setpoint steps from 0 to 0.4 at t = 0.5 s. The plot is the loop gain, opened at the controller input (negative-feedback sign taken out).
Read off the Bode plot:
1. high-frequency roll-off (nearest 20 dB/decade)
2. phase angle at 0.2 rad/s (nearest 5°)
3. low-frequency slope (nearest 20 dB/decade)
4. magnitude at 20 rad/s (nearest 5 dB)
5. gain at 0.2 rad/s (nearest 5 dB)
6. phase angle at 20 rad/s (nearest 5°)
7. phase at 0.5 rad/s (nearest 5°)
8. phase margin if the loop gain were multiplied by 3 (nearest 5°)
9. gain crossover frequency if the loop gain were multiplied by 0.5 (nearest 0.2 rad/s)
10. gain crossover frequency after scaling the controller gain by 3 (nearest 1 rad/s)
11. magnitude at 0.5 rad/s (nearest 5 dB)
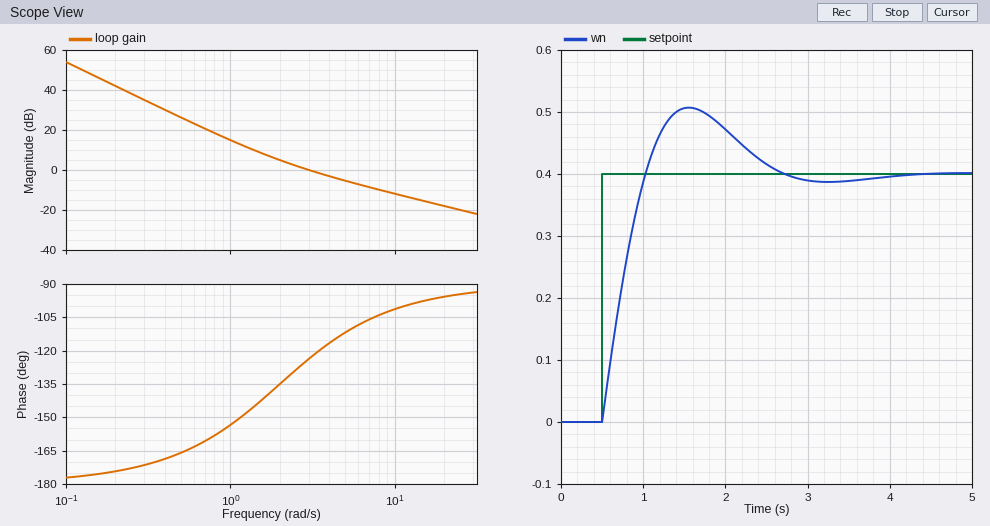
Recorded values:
-20 dB/decade
-175°
-40 dB/decade
-20 dB
40 dB
-95°
-165°
75°
1.8 rad/s
8 rad/s
25 dB
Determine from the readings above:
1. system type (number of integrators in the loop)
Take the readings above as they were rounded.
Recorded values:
2
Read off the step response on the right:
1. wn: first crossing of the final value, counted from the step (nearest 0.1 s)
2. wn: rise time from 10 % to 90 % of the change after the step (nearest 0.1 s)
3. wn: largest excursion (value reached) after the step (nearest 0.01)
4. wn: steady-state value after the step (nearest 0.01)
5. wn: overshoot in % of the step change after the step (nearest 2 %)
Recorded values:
0.5 s
0.4 s
0.51
0.40
26 %
